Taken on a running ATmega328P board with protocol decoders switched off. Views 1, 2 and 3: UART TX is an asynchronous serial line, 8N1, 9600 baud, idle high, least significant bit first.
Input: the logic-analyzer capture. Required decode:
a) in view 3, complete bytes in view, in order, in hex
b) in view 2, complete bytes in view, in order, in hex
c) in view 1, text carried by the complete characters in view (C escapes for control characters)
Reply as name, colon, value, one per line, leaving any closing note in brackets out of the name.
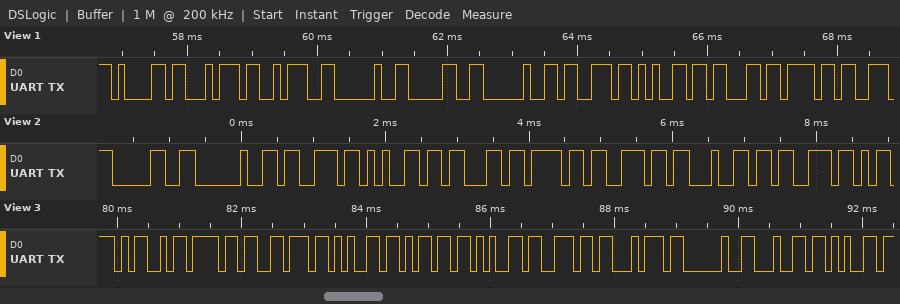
in view 3, complete bytes in view, in order, in hex: 0x4D 0x6F 0x76 0x65 0x6D 0x65 0x6E 0x74 0x20 0x64 0x65
in view 2, complete bytes in view, in order, in hex: 0x30 0x20 0x73 0x65 0x63 0x6F 0x6E 0x64 0x73
in view 1, text carried by the complete characters in view: "at: 0 seco"
